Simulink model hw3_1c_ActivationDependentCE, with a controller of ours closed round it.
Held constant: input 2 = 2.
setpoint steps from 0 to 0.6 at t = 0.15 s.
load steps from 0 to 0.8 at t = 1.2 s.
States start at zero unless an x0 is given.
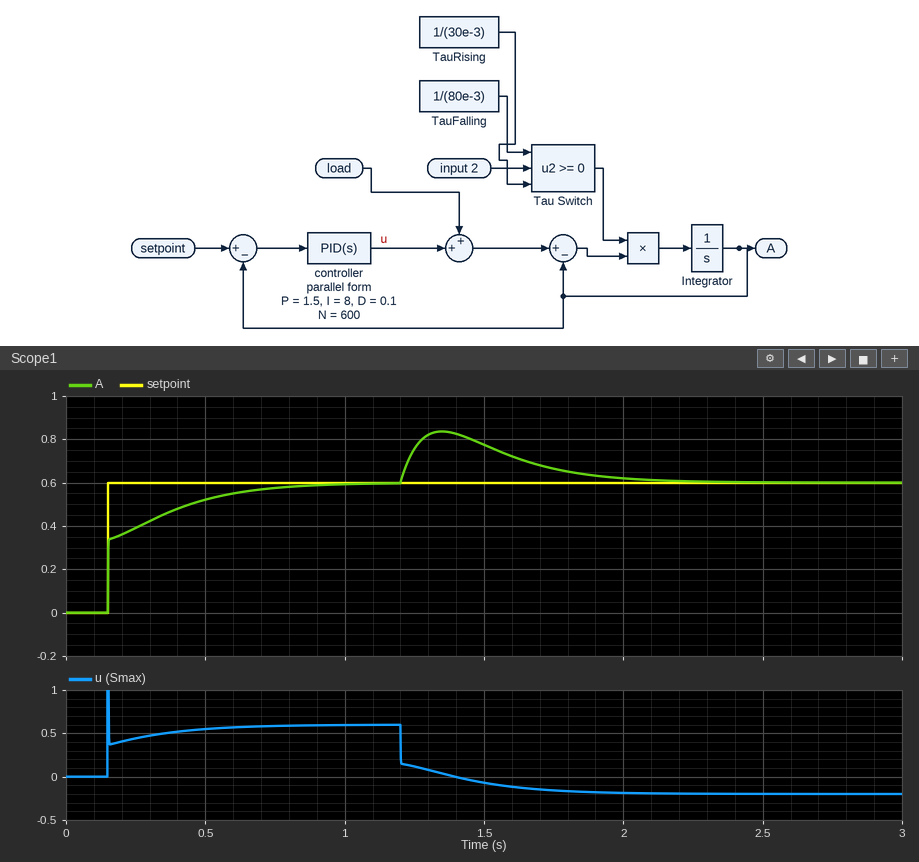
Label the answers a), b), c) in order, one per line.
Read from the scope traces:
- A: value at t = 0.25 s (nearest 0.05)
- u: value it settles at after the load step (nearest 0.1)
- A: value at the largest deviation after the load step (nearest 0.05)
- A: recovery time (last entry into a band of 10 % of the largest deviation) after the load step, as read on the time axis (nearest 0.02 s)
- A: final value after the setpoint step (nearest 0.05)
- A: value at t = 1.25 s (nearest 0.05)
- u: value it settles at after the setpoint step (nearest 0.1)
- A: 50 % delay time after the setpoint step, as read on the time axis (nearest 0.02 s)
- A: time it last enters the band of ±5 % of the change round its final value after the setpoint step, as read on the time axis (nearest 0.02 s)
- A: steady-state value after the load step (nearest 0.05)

a) 0.40
b) -0.2
c) 0.85
d) 1.96 s
e) 0.60
f) 0.75
g) 0.6
h) 0.16 s
i) 0.70 s
j) 0.60
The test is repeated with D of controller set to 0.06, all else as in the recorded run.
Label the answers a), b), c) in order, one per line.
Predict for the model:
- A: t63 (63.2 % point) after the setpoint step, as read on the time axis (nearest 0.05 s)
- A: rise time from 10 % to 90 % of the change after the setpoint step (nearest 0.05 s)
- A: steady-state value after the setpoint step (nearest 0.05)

a) 0.25 s
b) 0.40 s
c) 0.60
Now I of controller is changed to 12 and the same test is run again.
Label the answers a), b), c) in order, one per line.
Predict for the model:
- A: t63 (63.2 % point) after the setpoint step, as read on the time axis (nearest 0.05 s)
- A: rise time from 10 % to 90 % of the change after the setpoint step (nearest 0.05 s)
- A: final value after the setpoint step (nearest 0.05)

a) 0.20 s
b) 0.30 s
c) 0.60
